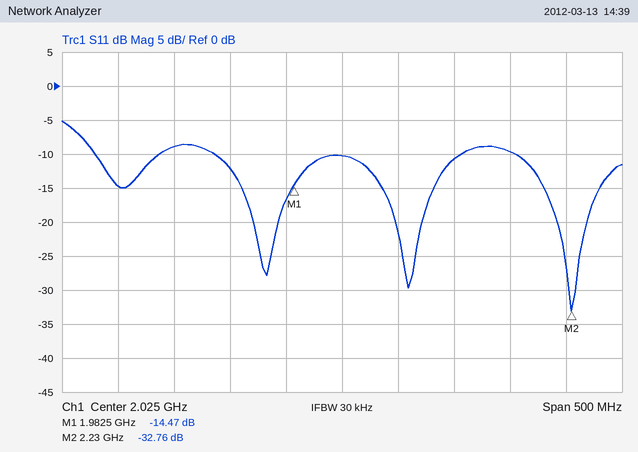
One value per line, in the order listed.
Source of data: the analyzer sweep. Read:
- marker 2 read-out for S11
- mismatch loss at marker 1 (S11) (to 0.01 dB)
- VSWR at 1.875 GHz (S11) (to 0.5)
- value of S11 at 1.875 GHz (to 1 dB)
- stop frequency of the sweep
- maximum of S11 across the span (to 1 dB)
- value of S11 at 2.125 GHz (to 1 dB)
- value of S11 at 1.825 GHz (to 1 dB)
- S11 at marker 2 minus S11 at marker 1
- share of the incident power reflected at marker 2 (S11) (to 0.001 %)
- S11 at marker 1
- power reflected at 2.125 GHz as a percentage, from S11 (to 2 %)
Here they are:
-32.76 dB
0.16 dB
2.0
-9 dB
2.275 GHz
-5 dB
-11 dB
-15 dB
-18.29 dB
0.053 %
-14.47 dB
8 %
